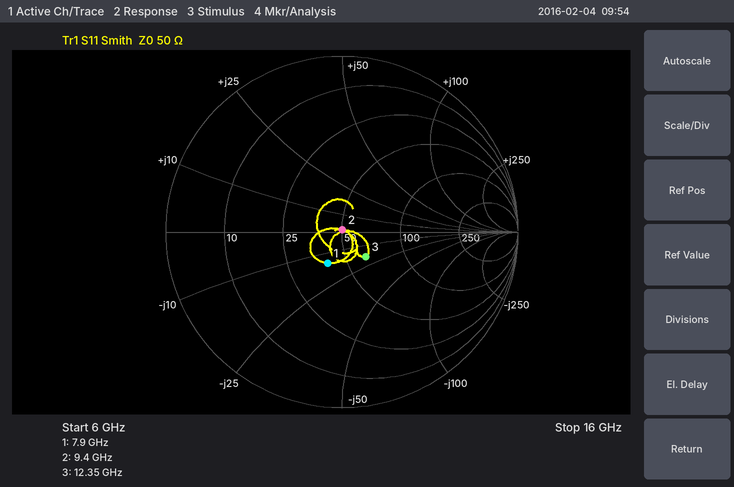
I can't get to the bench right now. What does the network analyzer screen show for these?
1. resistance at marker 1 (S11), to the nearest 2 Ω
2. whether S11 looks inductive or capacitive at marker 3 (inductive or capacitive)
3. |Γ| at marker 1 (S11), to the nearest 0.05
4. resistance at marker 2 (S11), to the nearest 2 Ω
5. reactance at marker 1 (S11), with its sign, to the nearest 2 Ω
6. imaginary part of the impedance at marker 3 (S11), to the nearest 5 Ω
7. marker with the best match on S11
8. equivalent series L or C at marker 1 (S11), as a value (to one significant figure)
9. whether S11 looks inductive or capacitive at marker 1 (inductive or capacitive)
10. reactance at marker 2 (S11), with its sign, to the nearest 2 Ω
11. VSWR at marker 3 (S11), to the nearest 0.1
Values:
40 Ω
capacitive
0.20
50 Ω
-14 Ω
-20 Ω
marker 2
1 pF
capacitive
+2 Ω
1.5
